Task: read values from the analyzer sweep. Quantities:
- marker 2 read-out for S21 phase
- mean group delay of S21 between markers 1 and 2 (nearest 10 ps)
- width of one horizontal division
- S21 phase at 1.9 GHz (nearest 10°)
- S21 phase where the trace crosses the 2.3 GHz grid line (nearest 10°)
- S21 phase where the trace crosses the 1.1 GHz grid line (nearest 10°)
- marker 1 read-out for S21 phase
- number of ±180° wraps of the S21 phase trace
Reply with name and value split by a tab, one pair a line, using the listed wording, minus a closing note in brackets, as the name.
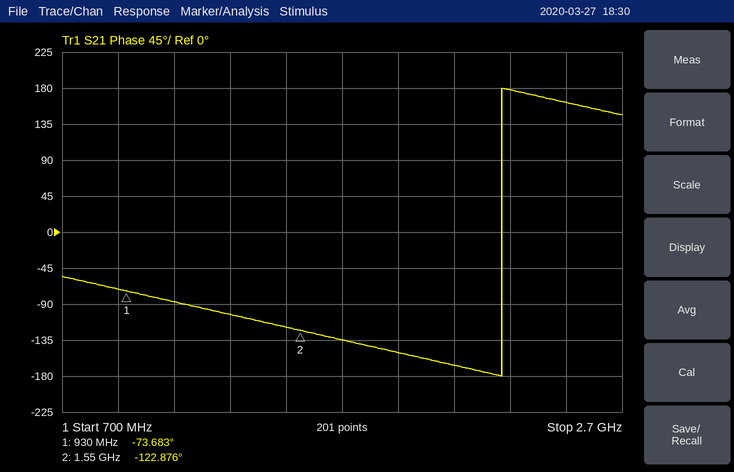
marker 2 read-out for S21 phase	-122.876°
mean group delay of S21 between markers 1 and 2	220 ps
width of one horizontal division	200 MHz
S21 phase at 1.9 GHz	-150°
S21 phase where the trace crosses the 2.3 GHz grid line	180°
S21 phase where the trace crosses the 1.1 GHz grid line	-90°
marker 1 read-out for S21 phase	-73.683°
number of ±180° wraps of the S21 phase trace	1
